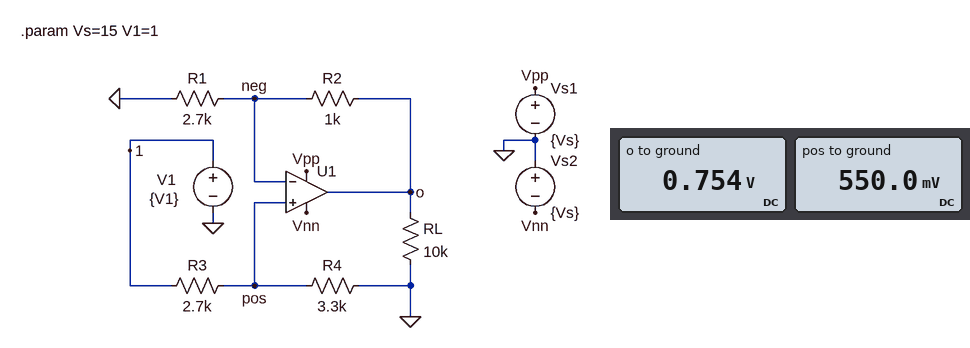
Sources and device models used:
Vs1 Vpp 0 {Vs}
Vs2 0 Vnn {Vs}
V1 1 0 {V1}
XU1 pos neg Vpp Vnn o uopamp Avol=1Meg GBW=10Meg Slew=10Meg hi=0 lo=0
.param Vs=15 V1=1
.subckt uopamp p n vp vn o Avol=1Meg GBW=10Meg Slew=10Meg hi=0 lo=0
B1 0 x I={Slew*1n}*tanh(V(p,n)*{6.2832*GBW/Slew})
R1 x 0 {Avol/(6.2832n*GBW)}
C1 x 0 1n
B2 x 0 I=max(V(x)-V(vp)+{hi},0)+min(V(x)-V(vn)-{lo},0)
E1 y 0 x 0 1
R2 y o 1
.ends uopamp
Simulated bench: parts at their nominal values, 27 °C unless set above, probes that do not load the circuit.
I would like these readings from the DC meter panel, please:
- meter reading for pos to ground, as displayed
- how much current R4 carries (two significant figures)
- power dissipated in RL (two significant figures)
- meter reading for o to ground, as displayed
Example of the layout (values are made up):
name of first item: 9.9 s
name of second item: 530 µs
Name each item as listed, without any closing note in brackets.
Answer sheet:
meter reading for pos to ground, as displayed: 550.0 mV
how much current R4 carries: 170 µA
power dissipated in RL: 57 µW
meter reading for o to ground, as displayed: 0.754 V
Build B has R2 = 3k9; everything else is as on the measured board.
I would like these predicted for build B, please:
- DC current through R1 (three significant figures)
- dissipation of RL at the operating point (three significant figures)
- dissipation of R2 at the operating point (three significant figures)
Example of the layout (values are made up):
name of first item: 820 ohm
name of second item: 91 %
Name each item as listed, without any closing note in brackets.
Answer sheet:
DC current through R1: 204 µA
dissipation of RL at the operating point: 181 µW
dissipation of R2 at the operating point: 162 µW
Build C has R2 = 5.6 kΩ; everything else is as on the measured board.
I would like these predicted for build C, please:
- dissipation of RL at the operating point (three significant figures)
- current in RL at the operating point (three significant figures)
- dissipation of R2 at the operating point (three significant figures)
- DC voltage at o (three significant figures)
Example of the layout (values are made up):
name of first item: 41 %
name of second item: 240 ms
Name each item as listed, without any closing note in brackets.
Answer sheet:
dissipation of RL at the operating point: 286 µW
current in RL at the operating point: 169 µA
dissipation of R2 at the operating point: 232 µW
DC voltage at o: 1.69 V
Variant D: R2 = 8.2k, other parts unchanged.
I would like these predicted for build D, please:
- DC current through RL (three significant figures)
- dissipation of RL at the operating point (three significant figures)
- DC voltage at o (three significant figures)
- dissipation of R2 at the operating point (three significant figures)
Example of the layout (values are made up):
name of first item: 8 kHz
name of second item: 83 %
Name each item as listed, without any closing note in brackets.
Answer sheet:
DC current through RL: 222 µA
dissipation of RL at the operating point: 493 µW
DC voltage at o: 2.22 V
dissipation of R2 at the operating point: 340 µW
